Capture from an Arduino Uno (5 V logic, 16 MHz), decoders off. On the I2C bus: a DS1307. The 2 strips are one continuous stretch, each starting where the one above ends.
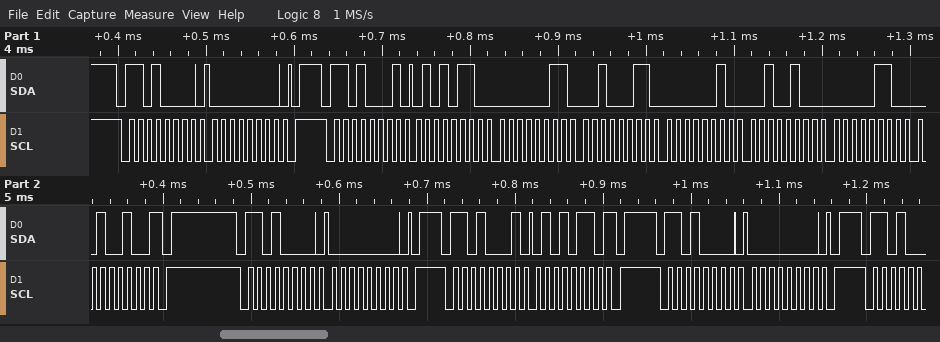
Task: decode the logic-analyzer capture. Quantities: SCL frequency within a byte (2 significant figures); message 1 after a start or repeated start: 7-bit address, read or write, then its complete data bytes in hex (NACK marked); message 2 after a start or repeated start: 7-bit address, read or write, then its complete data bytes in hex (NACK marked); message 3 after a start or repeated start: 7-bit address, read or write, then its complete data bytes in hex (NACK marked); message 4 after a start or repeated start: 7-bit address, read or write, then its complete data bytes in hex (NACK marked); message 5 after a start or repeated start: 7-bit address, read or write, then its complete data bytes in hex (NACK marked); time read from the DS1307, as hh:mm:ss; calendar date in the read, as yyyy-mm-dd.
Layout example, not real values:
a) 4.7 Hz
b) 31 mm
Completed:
a) 100 kHz
b) 0x68 write: 00
c) 0x68 read: 56 03 23 02 24 06 24 NACK
d) 0x68 write: 00
e) 0x68 read: 56 NACK
f) 0x68 write: 00
g) 23:03:56
h) 2024-06-24
